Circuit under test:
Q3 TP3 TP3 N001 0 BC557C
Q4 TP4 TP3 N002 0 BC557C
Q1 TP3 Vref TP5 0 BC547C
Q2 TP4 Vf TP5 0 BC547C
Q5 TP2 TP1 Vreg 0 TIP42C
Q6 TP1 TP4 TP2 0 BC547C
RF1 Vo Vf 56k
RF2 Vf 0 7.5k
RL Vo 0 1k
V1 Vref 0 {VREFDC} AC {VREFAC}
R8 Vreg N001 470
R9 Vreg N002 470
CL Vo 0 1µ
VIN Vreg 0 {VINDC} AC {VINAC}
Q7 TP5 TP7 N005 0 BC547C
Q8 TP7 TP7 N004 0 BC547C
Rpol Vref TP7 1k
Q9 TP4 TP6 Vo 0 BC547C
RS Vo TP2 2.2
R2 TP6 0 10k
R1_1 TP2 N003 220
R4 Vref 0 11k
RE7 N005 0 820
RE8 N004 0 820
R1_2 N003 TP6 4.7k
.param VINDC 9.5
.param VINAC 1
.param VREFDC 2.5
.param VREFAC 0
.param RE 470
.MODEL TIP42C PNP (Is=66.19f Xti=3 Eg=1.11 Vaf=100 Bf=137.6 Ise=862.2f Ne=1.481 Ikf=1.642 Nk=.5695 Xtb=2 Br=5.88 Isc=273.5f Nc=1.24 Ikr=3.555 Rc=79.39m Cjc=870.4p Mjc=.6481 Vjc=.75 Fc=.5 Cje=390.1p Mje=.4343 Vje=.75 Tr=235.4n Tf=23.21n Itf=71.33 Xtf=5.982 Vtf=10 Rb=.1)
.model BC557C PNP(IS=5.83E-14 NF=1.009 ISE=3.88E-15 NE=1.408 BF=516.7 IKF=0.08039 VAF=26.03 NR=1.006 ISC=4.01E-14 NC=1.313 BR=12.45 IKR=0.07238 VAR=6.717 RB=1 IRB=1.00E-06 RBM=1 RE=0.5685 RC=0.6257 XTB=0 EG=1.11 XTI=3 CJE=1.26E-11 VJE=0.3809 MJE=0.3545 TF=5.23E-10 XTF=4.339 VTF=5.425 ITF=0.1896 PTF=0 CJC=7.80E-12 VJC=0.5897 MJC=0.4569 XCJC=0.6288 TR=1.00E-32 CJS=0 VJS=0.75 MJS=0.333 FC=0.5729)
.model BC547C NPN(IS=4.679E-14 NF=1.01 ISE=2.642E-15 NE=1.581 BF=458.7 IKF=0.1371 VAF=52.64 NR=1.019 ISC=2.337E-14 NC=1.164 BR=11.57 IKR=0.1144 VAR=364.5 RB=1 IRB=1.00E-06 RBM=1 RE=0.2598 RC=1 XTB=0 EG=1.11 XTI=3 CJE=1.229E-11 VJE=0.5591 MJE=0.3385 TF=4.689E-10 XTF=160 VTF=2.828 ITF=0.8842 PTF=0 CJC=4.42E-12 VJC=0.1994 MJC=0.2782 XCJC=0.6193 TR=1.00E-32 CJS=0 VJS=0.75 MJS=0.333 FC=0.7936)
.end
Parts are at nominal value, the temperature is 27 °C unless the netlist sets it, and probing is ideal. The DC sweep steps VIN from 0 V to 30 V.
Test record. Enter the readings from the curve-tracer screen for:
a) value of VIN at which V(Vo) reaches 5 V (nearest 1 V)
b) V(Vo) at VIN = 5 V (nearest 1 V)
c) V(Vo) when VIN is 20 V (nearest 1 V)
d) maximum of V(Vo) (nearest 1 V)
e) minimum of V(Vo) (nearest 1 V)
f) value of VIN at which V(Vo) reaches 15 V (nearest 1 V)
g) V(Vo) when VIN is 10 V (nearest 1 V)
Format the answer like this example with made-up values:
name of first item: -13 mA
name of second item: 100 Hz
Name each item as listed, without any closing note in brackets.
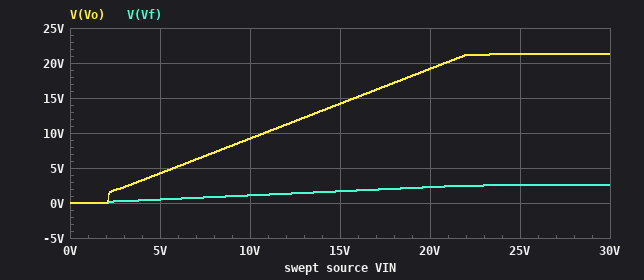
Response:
value of VIN at which V(Vo) reaches 5 V: 6 V
V(Vo) at VIN = 5 V: 4 V
V(Vo) when VIN is 20 V: 19 V
maximum of V(Vo): 21 V
minimum of V(Vo): 0 V
value of VIN at which V(Vo) reaches 15 V: 16 V
V(Vo) when VIN is 10 V: 9 V
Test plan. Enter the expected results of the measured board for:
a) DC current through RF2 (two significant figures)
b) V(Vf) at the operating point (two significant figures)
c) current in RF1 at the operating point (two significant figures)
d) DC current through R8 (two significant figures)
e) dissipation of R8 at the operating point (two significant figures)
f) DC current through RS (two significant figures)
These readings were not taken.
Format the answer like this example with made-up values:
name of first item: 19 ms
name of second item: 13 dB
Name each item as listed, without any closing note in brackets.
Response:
DC current through RF2: 140 µA
V(Vf) at the operating point: 1.0 V
current in RF1 at the operating point: 140 µA
DC current through R8: 580 µA
dissipation of R8 at the operating point: 160 µW
DC current through RS: 8.8 mA
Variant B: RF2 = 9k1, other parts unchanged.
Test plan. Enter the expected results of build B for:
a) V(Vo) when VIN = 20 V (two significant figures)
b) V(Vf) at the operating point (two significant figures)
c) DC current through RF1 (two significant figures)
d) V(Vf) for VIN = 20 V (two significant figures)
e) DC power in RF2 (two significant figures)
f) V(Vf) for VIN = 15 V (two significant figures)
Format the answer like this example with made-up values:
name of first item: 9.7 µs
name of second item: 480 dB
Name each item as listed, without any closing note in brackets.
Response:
V(Vo) when VIN = 20 V: 18 V
V(Vf) at the operating point: 1.2 V
DC current through RF1: 130 µA
V(Vf) for VIN = 20 V: 2.5 V
DC power in RF2: 160 µW
V(Vf) for VIN = 15 V: 2.0 V
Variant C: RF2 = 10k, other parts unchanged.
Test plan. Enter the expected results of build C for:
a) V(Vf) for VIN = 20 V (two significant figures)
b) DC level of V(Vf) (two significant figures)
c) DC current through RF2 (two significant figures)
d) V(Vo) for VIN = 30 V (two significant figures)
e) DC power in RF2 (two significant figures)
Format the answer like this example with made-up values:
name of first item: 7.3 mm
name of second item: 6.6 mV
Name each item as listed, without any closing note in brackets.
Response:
V(Vf) for VIN = 20 V: 2.5 V
DC level of V(Vf): 1.3 V
DC current through RF2: 130 µA
V(Vo) for VIN = 30 V: 17 V
DC power in RF2: 170 µW
